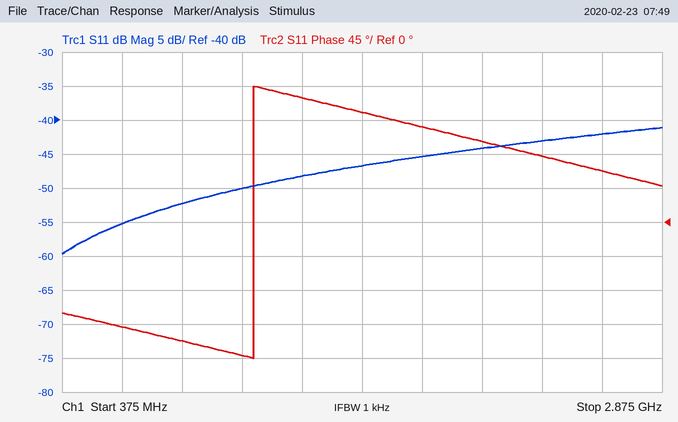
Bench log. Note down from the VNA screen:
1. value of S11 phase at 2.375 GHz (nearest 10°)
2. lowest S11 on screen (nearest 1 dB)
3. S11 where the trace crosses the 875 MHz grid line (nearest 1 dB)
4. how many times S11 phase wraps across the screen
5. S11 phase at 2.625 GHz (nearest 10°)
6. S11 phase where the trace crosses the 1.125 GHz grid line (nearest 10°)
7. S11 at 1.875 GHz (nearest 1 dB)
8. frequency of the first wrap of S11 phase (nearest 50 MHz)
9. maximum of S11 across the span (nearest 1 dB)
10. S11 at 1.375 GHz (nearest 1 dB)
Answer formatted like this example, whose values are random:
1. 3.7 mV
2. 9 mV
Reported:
1. 90°
2. -60 dB
3. -52 dB
4. 1
5. 70°
6. -180°
7. -45 dB
8. 1.15 GHz
9. -41 dB
10. -48 dB
